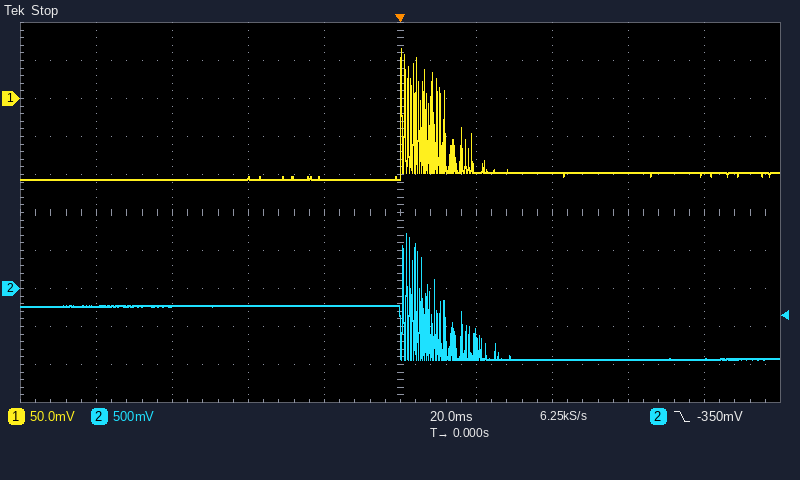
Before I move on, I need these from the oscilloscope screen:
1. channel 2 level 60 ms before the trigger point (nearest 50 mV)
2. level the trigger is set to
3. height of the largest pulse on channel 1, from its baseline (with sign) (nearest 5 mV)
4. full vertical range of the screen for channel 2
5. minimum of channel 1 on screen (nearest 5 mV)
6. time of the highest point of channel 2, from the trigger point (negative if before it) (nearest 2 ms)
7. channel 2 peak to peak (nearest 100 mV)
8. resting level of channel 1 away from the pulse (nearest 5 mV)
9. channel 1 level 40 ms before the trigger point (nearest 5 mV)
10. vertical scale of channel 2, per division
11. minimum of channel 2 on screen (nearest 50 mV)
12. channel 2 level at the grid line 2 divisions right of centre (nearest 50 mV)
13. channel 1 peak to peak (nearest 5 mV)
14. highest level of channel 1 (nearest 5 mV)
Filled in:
-250 mV
-350 mV
+170 mV
5 V
-105 mV
+2 ms
1.70 V
-105 mV
-105 mV
500 mV
-950 mV
-950 mV
170 mV
65 mV
